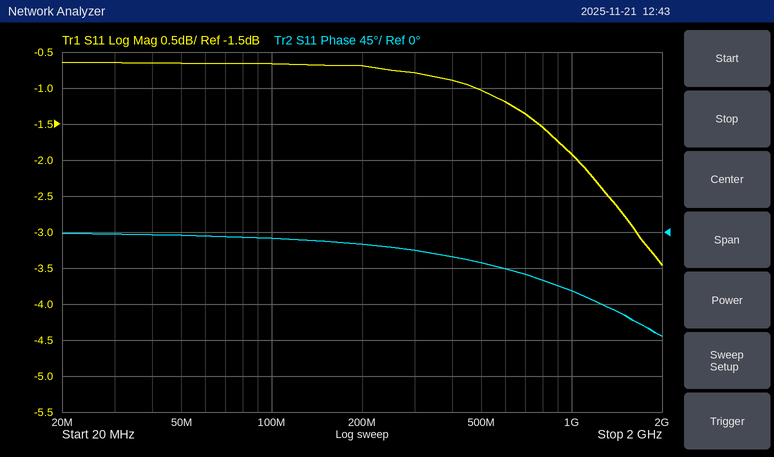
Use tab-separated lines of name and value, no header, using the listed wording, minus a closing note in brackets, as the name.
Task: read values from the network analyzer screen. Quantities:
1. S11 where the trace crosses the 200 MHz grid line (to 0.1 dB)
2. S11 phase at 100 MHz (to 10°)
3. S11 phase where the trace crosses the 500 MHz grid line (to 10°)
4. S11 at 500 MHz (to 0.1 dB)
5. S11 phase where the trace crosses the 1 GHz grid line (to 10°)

S11 where the trace crosses the 200 MHz grid line	-0.7 dB
S11 phase at 100 MHz	-10°
S11 phase where the trace crosses the 500 MHz grid line	-40°
S11 at 500 MHz	-1.0 dB
S11 phase where the trace crosses the 1 GHz grid line	-70°
